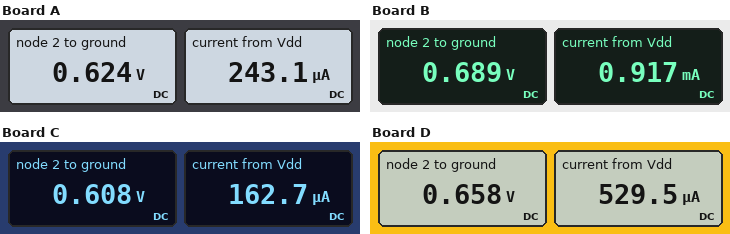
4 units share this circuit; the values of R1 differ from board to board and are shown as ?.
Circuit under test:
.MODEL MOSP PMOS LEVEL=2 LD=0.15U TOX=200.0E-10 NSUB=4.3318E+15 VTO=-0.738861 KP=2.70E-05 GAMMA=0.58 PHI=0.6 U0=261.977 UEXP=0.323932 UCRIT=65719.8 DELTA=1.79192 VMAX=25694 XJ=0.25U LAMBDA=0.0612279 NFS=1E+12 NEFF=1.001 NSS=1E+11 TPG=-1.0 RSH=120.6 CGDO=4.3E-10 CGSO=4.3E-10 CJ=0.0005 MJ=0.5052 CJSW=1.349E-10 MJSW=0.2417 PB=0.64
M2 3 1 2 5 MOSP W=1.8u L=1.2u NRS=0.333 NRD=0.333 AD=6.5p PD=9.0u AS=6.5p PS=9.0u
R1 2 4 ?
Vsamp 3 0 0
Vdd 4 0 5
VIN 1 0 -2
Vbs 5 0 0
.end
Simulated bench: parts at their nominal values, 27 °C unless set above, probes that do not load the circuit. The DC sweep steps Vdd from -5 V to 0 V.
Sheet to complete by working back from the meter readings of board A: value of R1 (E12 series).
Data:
18 kΩ
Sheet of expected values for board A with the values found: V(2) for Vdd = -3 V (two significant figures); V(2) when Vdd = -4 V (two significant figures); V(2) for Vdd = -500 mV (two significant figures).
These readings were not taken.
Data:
-2.5 V
-3.4 V
-280 mV
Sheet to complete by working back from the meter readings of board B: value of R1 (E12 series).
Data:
4.7 kΩ
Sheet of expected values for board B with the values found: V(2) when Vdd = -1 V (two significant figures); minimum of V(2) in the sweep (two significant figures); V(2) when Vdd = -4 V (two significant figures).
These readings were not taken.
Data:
-880 mV
-4.8 V
-3.8 V
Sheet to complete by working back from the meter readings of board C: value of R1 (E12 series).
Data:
27 kΩ
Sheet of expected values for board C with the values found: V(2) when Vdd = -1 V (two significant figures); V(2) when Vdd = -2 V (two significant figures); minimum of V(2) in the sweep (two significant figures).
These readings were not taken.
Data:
-480 mV
-1.3 V
-4.1 V
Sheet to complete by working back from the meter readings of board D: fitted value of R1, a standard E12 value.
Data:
8.2 kΩ
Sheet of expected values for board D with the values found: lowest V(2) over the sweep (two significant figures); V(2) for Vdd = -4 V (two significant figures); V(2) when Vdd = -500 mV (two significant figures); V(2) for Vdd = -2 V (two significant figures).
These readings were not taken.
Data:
-4.7 V
-3.7 V
-370 mV
-1.8 V
